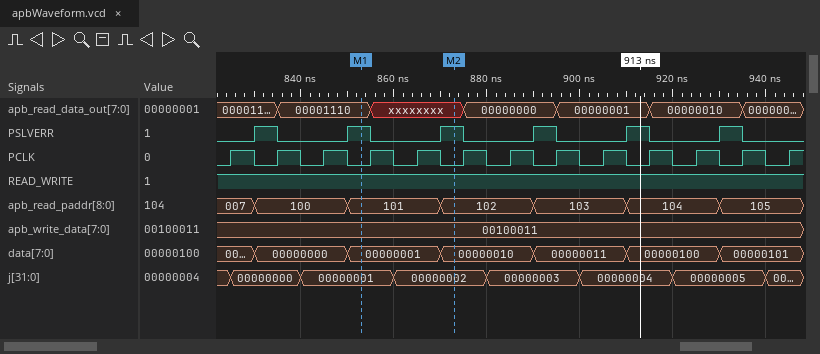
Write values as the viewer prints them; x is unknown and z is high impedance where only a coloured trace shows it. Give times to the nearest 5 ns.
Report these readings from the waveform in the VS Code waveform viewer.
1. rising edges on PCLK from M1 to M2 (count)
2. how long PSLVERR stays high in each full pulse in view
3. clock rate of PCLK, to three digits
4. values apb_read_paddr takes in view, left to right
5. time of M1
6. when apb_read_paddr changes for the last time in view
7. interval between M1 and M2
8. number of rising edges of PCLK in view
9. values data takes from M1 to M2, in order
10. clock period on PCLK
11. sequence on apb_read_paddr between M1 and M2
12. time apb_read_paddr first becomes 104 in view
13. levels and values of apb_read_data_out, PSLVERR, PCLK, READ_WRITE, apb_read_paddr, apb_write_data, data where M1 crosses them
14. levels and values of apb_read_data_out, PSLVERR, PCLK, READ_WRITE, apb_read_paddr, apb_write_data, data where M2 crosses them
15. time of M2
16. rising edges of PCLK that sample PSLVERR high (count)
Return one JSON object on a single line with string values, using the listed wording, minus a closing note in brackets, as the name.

{"rising edges on PCLK from M1 to M2": "2", "how long PSLVERR stays high in each full pulse in view": "5 ns, 5 ns, 5 ns, 5 ns, 5 ns, 5 ns", "clock rate of PCLK, to three digits": "100 MHz", "values apb_read_paddr takes in view, left to right": "007, 100, 101, 102, 103, 104, 105", "time of M1": "855 ns", "when apb_read_paddr changes for the last time in view": "930 ns", "interval between M1 and M2": "20 ns", "number of rising edges of PCLK in view": "13", "values data takes from M1 to M2, in order": "00000001, 00000010", "clock period on PCLK": "10 ns", "sequence on apb_read_paddr between M1 and M2": "101, 102", "time apb_read_paddr first becomes 104 in view": "910 ns", "levels and values of apb_read_data_out, PSLVERR, PCLK, READ_WRITE, apb_read_paddr, apb_write_data, data where M1 crosses them": "apb_read_data_out=00001110, PSLVERR=1, PCLK=0, READ_WRITE=1, apb_read_paddr=101, apb_write_data=00100011, data=00000001", "levels and values of apb_read_data_out, PSLVERR, PCLK, READ_WRITE, apb_read_paddr, apb_write_data, data where M2 crosses them": "apb_read_data_out=xxxxxxxx, PSLVERR=1, PCLK=0, READ_WRITE=1, apb_read_paddr=102, apb_write_data=00100011, data=00000010", "time of M2": "875 ns", "rising edges of PCLK that sample PSLVERR high": "6"}
